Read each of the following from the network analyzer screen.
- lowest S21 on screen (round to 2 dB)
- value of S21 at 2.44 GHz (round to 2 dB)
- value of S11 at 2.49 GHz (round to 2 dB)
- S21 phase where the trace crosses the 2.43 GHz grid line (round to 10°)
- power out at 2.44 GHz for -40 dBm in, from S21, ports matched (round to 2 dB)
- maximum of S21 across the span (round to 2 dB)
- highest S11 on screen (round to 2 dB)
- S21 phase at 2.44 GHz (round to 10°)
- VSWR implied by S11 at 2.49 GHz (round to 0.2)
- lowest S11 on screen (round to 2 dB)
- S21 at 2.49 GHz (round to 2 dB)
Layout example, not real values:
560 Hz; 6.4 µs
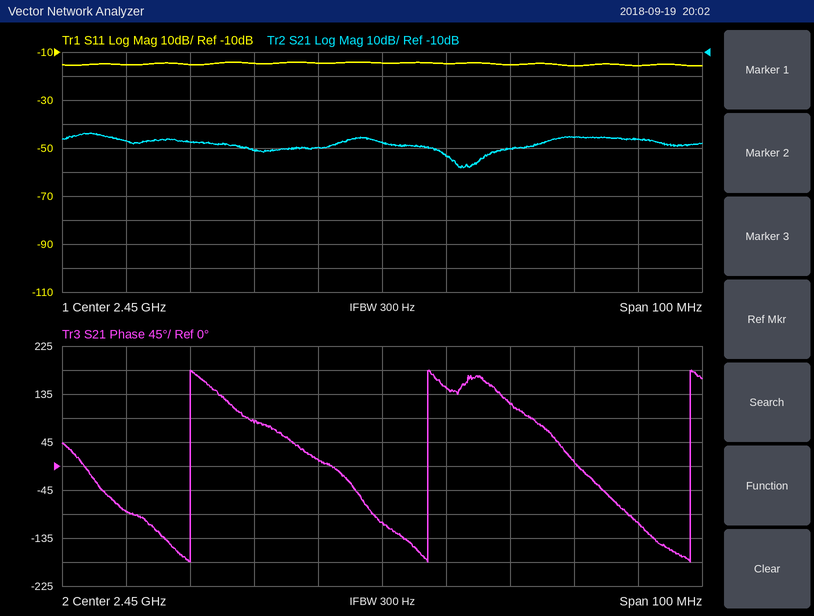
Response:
-58 dB; -50 dB; -16 dB; 80°; -90 dBm; -44 dB; -14 dB; 10°; 1.4; -16 dB; -46 dB
